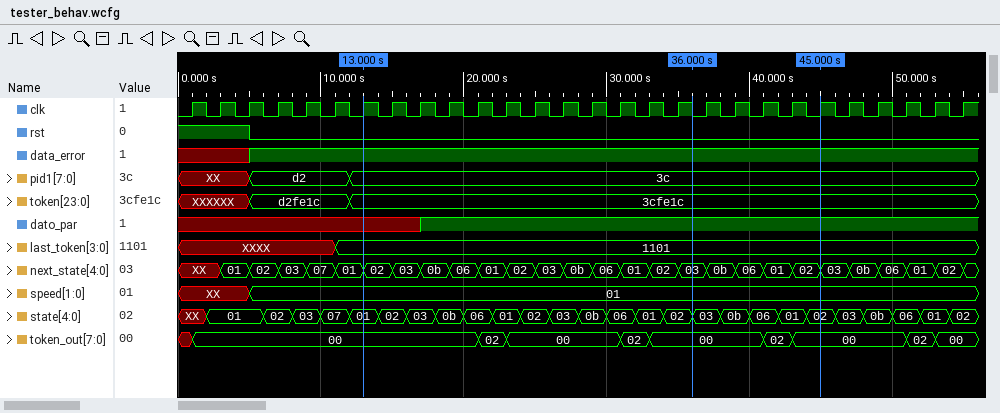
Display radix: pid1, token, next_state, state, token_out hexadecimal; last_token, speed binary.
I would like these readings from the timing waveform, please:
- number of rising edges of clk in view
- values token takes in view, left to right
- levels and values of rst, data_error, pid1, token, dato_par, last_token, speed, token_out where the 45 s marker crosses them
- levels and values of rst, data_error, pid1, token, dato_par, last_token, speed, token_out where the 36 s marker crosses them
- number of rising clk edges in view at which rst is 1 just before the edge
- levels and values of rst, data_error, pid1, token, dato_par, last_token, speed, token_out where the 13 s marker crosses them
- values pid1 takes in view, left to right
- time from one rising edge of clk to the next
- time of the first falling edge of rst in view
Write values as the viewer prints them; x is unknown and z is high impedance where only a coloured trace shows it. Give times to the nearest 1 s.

28
XXXXXX, d2fe1c, 3cfe1c
rst=0, data_error=1, pid1=3c, token=3cfe1c, dato_par=1, last_token=1101, speed=01, token_out=00
rst=0, data_error=1, pid1=3c, token=3cfe1c, dato_par=1, last_token=1101, speed=01, token_out=00
3
rst=0, data_error=1, pid1=3c, token=3cfe1c, dato_par=x, last_token=1101, speed=01, token_out=00
XX, d2, 3c
2 s
5 s
